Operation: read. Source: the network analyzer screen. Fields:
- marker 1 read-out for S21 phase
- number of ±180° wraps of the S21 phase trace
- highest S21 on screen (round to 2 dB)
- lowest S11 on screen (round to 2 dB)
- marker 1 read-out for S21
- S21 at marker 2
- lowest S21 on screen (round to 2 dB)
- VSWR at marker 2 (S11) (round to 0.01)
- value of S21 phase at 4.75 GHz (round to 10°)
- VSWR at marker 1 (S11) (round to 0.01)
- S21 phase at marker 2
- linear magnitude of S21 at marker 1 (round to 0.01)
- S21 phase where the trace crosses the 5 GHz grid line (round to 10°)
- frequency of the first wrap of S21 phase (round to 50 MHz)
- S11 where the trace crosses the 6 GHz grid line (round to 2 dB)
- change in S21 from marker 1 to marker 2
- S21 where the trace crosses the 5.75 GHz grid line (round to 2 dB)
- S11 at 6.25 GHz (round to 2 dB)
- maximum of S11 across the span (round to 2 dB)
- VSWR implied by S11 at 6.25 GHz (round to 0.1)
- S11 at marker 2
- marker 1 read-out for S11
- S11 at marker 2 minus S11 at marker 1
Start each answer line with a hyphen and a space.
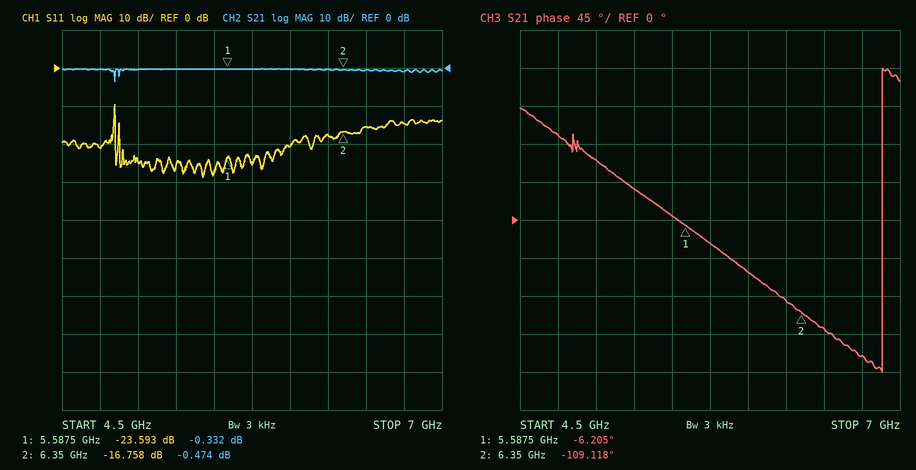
- -6.205°
- 1
- 0 dB
- -28 dB
- -0.332 dB
- -0.474 dB
- -4 dB
- 1.34
- 100°
- 1.14
- -109.118°
- 0.96
- 70°
- 6.90 GHz
- -20 dB
- -0.142 dB
- 0 dB
- -18 dB
- -10 dB
- 1.3
- -16.758 dB
- -23.593 dB
- 6.835 dB
